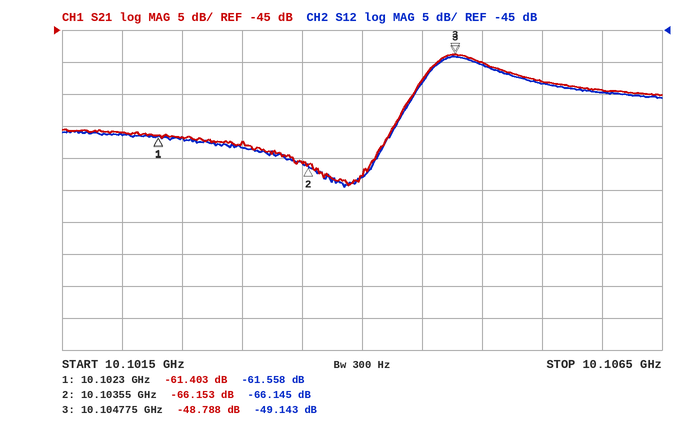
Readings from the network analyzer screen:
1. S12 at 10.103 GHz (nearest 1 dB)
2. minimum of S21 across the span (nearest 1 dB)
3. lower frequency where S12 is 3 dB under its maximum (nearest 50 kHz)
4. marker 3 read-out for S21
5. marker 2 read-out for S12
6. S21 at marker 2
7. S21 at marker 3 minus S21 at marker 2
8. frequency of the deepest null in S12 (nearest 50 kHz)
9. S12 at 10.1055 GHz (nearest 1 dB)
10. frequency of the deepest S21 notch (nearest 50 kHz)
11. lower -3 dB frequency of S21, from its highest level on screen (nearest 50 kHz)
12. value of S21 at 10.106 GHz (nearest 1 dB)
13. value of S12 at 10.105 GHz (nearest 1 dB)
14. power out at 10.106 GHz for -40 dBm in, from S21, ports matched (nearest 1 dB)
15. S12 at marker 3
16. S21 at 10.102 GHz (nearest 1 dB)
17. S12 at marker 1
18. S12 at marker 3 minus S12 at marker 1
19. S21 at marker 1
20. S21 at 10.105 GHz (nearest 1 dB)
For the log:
-63 dB
-69 dB
10.10455 GHz
-48.788 dB
-66.145 dB
-66.153 dB
17.365 dB
10.10385 GHz
-53 dB
10.10390 GHz
10.10455 GHz
-54 dB
-50 dB
-94 dBm
-49.143 dB
-61 dB
-61.558 dB
12.415 dB
-61.403 dB
-50 dB
